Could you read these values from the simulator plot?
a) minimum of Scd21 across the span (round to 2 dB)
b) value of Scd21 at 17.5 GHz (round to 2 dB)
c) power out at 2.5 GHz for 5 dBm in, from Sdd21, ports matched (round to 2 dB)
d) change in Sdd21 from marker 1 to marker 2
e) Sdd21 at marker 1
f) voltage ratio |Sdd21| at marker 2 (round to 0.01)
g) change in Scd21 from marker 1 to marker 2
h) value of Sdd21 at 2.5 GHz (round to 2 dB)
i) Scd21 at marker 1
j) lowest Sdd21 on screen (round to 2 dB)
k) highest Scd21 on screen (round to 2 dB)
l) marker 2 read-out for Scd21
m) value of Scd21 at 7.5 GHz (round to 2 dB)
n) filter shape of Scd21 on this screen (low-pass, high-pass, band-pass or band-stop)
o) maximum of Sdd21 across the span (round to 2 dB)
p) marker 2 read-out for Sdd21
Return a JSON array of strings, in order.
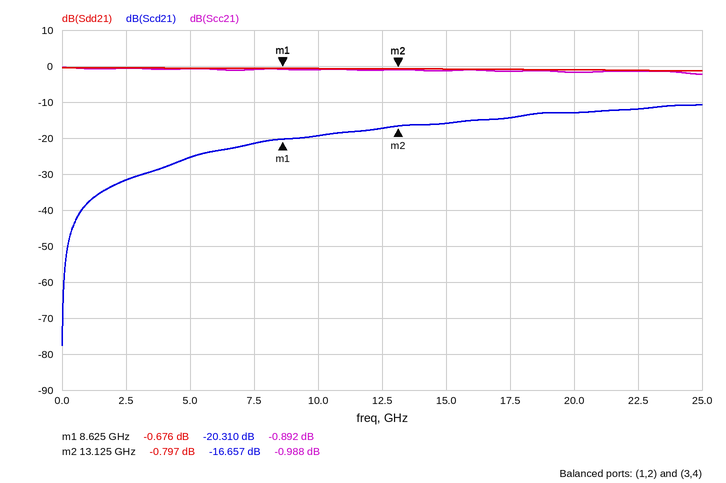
["-78 dB", "-14 dB", "4 dBm", "-0.121 dB", "-0.676 dB", "0.91", "3.653 dB", "0 dB", "-20.310 dB", "-2 dB", "-10 dB", "-16.657 dB", "-22 dB", "high-pass", "0 dB", "-0.797 dB"]
